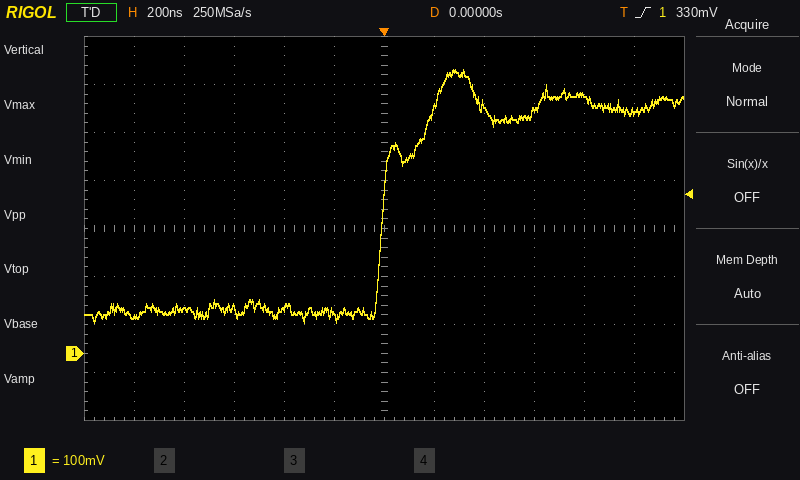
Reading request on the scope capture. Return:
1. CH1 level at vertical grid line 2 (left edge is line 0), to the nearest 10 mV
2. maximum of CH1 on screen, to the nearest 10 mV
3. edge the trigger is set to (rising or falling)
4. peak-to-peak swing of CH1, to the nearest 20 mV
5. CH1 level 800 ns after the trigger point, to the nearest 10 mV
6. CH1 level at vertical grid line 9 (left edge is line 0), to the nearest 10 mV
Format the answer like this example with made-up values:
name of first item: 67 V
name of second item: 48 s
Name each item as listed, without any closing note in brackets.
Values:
CH1 level at vertical grid line 2 (left edge is line 0), to the nearest 10 mV: 90 mV
maximum of CH1 on screen, to the nearest 10 mV: 590 mV
edge the trigger is set to: rising
peak-to-peak swing of CH1, to the nearest 20 mV: 520 mV
CH1 level 800 ns after the trigger point, to the nearest 10 mV: 540 mV
CH1 level at vertical grid line 9 (left edge is line 0), to the nearest 10 mV: 500 mV
